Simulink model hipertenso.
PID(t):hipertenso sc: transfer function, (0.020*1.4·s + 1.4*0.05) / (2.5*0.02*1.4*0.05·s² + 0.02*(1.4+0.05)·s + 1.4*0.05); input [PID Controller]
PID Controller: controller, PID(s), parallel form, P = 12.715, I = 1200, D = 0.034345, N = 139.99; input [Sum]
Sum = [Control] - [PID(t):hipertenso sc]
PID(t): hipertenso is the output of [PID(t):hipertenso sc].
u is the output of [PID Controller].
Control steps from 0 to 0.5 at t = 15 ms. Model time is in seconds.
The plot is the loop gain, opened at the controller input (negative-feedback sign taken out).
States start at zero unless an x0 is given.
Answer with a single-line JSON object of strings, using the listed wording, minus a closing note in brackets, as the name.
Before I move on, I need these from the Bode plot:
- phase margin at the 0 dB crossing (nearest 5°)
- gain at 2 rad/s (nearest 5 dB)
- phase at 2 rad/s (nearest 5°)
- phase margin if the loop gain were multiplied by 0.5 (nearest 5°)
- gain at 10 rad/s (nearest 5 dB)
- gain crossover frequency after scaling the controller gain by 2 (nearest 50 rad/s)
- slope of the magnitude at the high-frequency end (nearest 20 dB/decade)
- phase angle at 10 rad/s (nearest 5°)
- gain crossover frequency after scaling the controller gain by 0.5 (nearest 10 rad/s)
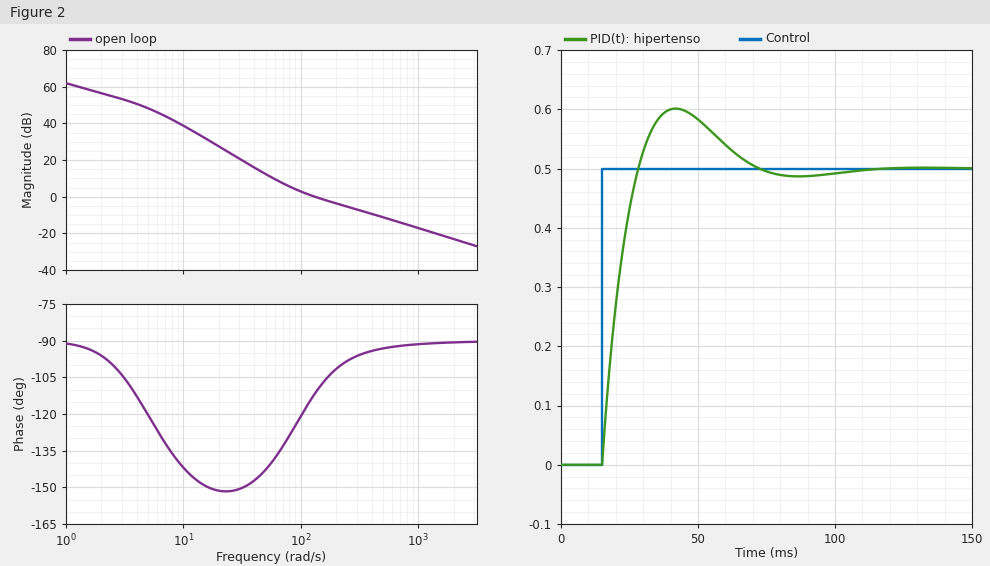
{"phase margin at the 0 dB crossing": "70°", "gain at 2 rad/s": "55 dB", "phase at 2 rad/s": "-95°", "phase margin if the loop gain were multiplied by 0.5": "50°", "gain at 10 rad/s": "40 dB", "gain crossover frequency after scaling the controller gain by 2": "250 rad/s", "slope of the magnitude at the high-frequency end": "-20 dB/decade", "phase angle at 10 rad/s": "-140°", "gain crossover frequency after scaling the controller gain by 0.5": "80 rad/s"}
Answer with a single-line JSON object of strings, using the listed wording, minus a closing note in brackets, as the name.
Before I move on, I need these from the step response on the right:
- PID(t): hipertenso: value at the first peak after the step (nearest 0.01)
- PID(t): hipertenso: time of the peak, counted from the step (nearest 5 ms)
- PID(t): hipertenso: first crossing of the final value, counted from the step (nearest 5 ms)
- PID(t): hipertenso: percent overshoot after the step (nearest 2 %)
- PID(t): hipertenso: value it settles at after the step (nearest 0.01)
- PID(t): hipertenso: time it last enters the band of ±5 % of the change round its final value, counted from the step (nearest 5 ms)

{"PID(t): hipertenso: value at the first peak after the step": "0.60", "PID(t): hipertenso: time of the peak, counted from the step": "25 ms", "PID(t): hipertenso: first crossing of the final value, counted from the step": "15 ms", "PID(t): hipertenso: percent overshoot after the step": "20 %", "PID(t): hipertenso: value it settles at after the step": "0.50", "PID(t): hipertenso: time it last enters the band of ±5 % of the change round its final value, counted from the step": "50 ms"}
